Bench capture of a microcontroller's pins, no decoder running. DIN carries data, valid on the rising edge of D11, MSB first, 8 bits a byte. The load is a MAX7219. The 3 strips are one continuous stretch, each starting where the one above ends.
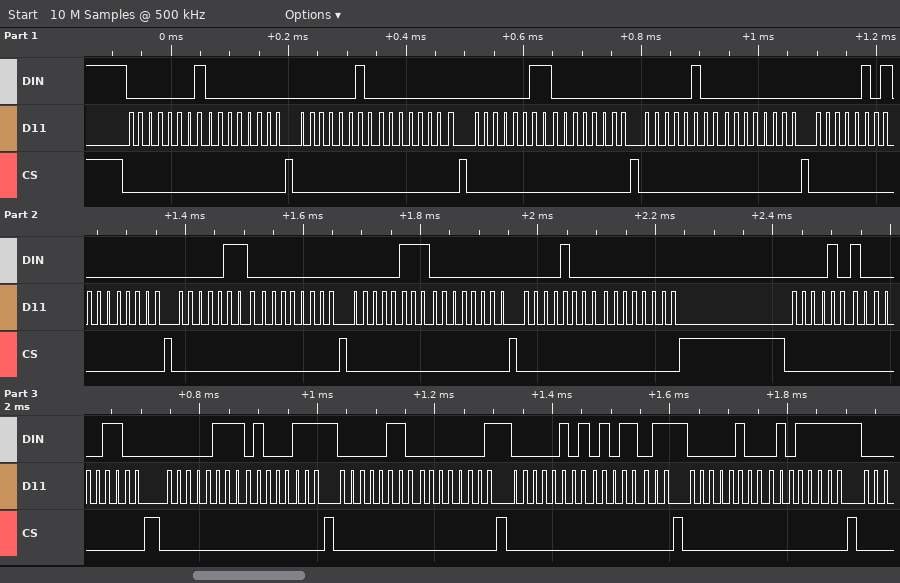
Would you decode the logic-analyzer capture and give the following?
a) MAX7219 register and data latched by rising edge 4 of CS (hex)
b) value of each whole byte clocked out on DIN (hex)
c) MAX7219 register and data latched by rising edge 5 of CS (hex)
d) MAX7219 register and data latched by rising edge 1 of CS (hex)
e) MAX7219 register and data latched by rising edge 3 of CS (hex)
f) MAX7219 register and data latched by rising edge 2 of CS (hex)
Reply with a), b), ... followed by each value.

a) register 0x4, data 0x00
b) 0x01 0x00 0x02 0x00 0x03 0x00 0x04 0x00 0x05 0x00 0x06 0x00 0x07 0x00 0x08 0x00 0x0A 0x0C 0x07 0x47 0x06 0x01 0x05 0x5B 0x04 0x5F
c) register 0x5, data 0x00
d) register 0x1, data 0x00
e) register 0x3, data 0x00
f) register 0x2, data 0x00
